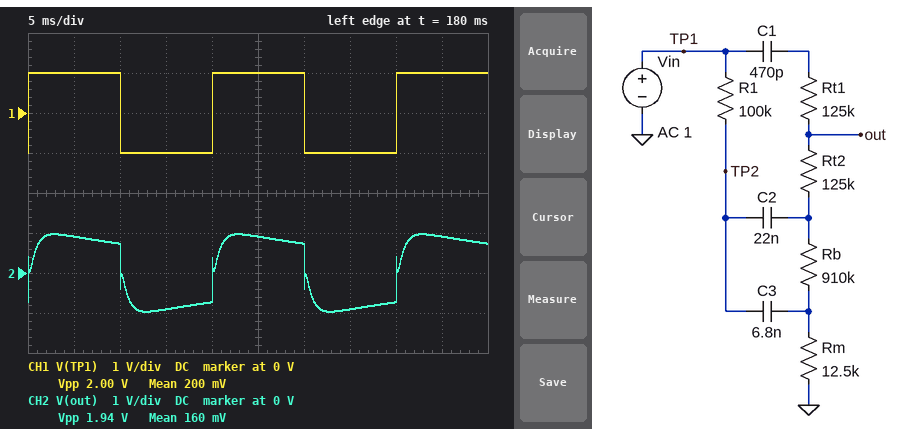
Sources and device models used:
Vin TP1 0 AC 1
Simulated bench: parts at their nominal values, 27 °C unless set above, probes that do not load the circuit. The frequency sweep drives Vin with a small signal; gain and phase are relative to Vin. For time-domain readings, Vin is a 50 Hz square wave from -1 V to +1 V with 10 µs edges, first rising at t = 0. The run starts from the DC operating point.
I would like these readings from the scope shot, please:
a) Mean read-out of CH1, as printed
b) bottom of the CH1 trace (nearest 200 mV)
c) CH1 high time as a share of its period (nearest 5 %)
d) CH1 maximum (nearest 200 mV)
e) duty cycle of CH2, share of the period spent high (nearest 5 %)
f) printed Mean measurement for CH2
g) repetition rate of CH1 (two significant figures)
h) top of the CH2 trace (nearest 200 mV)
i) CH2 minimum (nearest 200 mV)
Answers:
200 mV
-1.0 V
50 %
1.0 V
50 %
160 mV
50 Hz
1.0 V
-1.0 V
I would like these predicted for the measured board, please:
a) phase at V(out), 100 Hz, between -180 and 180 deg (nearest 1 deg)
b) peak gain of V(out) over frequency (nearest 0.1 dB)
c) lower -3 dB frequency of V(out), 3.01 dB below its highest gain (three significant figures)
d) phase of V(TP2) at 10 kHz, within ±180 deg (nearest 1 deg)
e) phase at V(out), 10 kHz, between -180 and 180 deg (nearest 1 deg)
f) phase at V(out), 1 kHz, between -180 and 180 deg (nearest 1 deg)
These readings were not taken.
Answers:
-15 deg
-1.1 dB
6.51 Hz
-7 deg
5 deg
9 deg
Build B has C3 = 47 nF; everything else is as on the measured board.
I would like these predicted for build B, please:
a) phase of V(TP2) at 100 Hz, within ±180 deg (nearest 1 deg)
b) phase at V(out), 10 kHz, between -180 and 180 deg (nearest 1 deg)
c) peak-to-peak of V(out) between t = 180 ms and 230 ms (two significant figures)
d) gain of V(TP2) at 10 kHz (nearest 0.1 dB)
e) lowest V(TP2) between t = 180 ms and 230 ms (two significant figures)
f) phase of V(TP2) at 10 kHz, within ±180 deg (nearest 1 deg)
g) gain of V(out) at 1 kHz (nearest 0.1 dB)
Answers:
-50 deg
6 deg
1.3 V
-16.6 dB
-730 mV
1 deg
-9.2 dB
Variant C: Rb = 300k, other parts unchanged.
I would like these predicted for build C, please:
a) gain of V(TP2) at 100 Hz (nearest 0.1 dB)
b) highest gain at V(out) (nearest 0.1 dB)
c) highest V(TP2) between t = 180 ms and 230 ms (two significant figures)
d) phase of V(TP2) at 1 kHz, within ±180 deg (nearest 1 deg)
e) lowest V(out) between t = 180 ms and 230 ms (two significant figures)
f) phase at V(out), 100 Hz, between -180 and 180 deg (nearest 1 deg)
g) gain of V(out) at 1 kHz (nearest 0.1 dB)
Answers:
-3.0 dB
-2.9 dB
860 mV
-38 deg
-920 mV
-5 deg
-9.8 dB
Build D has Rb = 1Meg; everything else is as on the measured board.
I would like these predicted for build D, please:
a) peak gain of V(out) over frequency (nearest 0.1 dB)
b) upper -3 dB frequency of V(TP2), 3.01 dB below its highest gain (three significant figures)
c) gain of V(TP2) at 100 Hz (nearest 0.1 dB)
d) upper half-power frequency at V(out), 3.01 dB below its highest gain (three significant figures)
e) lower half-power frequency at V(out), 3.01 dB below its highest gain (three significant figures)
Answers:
-1.0 dB
181 Hz
-1.6 dB
214 Hz
6.01 Hz
